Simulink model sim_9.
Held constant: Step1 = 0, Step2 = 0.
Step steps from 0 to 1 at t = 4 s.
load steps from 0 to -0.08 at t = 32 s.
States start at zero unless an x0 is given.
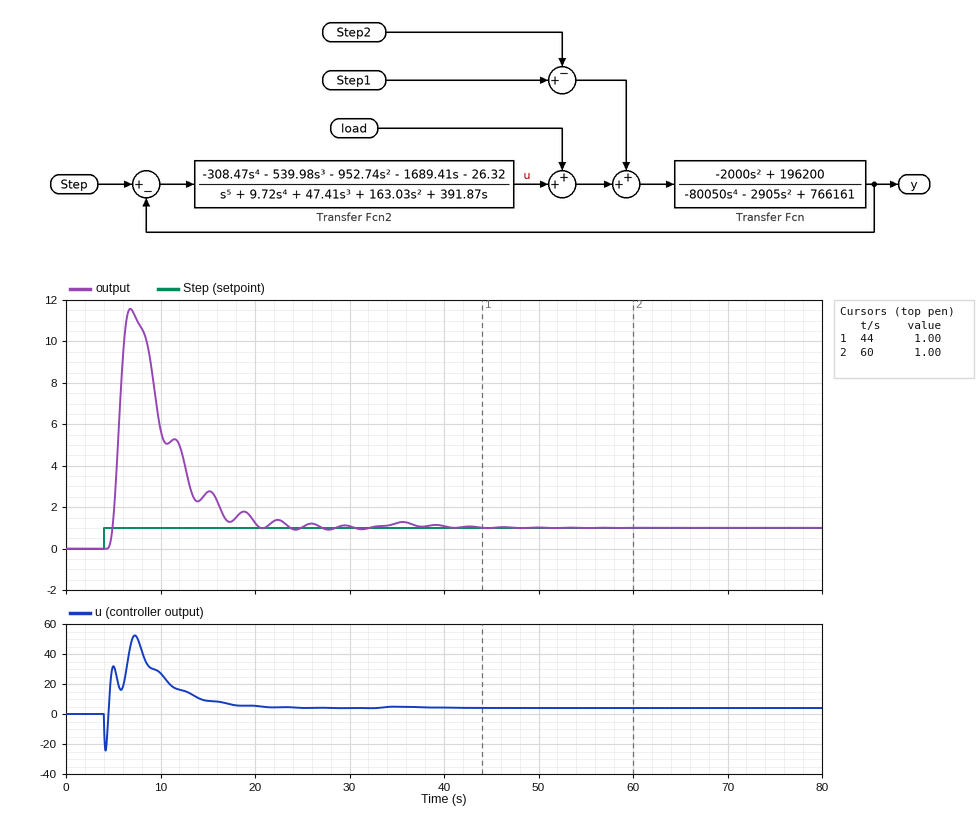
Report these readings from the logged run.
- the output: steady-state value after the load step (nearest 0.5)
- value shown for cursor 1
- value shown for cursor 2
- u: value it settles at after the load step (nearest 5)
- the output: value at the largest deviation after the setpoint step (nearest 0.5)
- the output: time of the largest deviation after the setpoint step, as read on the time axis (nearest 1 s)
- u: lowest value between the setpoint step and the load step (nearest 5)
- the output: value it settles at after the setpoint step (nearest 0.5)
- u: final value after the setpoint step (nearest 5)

1.0
1.00
1.00
5
11.5
7 s
-25
1.0
5
